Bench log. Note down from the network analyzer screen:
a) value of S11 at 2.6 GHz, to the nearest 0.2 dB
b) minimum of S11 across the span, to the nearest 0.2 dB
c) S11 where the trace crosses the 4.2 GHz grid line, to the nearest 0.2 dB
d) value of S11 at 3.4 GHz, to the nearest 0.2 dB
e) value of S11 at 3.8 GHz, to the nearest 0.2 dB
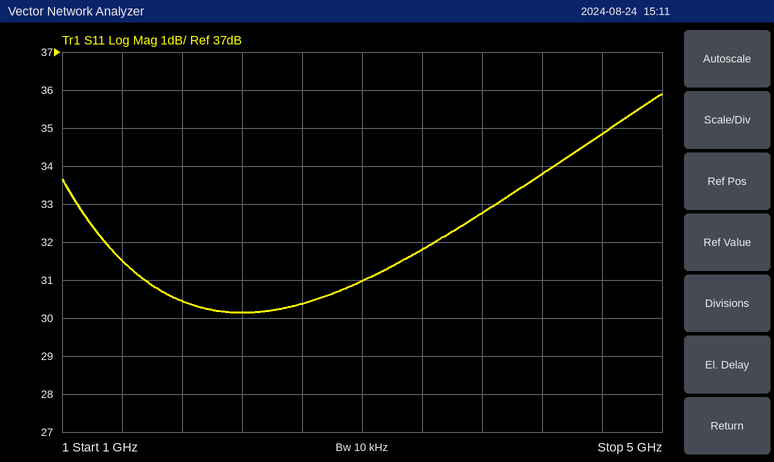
30.4 dB
30.2 dB
33.8 dB
31.8 dB
32.8 dB
